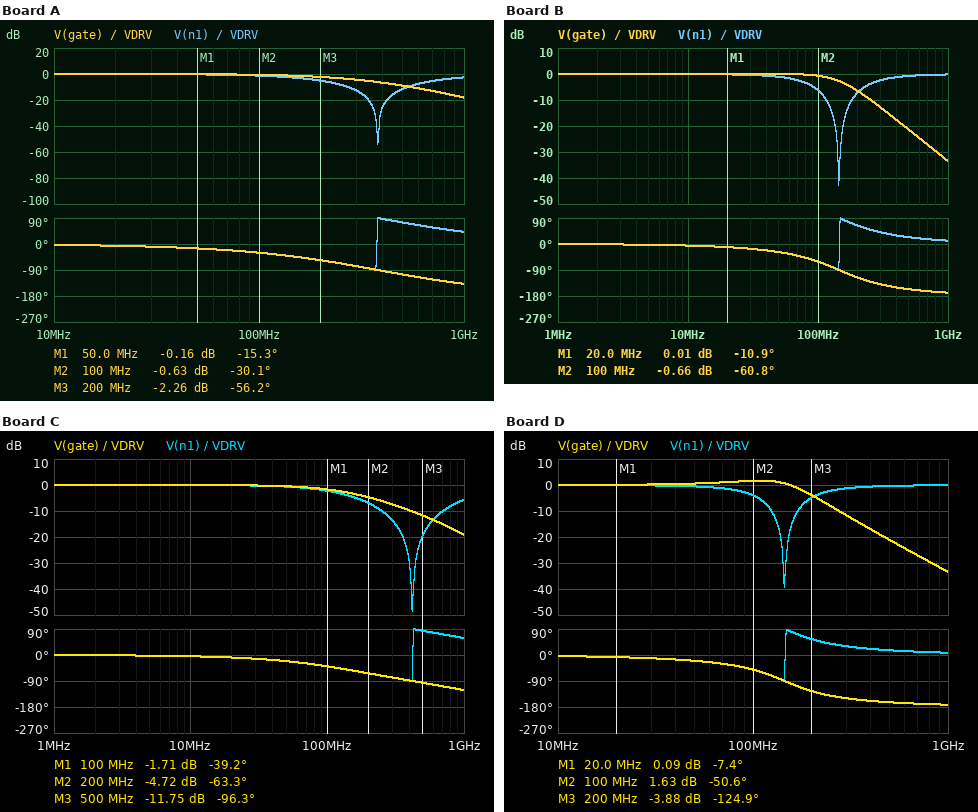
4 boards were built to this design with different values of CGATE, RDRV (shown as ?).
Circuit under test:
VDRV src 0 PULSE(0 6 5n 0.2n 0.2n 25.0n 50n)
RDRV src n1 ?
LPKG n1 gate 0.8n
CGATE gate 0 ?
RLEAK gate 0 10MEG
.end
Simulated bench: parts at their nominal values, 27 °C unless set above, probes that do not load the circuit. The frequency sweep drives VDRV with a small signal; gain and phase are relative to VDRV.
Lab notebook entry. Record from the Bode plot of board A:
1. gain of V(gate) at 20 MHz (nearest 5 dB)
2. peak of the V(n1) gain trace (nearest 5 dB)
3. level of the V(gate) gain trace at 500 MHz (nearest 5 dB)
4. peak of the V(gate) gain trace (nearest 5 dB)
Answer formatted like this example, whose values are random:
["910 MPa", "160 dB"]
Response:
["0 dB", "0 dB", "-10 dB", "0 dB"]
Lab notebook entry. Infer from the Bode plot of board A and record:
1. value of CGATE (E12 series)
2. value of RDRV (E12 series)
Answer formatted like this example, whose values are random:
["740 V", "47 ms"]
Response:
["220 pF", "3.9 Ω"]
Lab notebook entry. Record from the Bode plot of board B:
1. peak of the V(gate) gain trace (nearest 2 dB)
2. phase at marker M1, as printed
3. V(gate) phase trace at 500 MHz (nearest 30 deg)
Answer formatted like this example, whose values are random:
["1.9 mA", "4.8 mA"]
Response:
["0 dB", "-10.9 deg", "-150 deg"]
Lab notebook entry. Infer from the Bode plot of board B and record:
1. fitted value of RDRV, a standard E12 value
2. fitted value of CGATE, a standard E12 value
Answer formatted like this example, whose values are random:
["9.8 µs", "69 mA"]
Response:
["1 Ω", "1.5 nF"]
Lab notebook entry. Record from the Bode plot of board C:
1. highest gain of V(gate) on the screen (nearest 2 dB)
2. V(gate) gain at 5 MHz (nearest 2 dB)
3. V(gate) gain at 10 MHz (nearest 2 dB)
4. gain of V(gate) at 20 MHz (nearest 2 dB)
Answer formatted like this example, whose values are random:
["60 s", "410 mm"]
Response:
["0 dB", "0 dB", "0 dB", "0 dB"]
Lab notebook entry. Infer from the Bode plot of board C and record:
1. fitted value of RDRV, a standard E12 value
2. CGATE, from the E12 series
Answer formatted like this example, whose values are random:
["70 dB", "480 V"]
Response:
["6.8 Ω", "180 pF"]
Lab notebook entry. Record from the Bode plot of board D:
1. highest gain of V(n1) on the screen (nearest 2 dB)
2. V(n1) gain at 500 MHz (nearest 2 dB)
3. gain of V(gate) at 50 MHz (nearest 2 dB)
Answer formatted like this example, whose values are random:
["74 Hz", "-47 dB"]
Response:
["0 dB", "0 dB", "0 dB"]
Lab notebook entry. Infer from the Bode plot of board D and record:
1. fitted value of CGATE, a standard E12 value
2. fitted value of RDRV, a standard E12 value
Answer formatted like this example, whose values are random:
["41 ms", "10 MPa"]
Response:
["1.5 nF", "0.68 Ω"]
